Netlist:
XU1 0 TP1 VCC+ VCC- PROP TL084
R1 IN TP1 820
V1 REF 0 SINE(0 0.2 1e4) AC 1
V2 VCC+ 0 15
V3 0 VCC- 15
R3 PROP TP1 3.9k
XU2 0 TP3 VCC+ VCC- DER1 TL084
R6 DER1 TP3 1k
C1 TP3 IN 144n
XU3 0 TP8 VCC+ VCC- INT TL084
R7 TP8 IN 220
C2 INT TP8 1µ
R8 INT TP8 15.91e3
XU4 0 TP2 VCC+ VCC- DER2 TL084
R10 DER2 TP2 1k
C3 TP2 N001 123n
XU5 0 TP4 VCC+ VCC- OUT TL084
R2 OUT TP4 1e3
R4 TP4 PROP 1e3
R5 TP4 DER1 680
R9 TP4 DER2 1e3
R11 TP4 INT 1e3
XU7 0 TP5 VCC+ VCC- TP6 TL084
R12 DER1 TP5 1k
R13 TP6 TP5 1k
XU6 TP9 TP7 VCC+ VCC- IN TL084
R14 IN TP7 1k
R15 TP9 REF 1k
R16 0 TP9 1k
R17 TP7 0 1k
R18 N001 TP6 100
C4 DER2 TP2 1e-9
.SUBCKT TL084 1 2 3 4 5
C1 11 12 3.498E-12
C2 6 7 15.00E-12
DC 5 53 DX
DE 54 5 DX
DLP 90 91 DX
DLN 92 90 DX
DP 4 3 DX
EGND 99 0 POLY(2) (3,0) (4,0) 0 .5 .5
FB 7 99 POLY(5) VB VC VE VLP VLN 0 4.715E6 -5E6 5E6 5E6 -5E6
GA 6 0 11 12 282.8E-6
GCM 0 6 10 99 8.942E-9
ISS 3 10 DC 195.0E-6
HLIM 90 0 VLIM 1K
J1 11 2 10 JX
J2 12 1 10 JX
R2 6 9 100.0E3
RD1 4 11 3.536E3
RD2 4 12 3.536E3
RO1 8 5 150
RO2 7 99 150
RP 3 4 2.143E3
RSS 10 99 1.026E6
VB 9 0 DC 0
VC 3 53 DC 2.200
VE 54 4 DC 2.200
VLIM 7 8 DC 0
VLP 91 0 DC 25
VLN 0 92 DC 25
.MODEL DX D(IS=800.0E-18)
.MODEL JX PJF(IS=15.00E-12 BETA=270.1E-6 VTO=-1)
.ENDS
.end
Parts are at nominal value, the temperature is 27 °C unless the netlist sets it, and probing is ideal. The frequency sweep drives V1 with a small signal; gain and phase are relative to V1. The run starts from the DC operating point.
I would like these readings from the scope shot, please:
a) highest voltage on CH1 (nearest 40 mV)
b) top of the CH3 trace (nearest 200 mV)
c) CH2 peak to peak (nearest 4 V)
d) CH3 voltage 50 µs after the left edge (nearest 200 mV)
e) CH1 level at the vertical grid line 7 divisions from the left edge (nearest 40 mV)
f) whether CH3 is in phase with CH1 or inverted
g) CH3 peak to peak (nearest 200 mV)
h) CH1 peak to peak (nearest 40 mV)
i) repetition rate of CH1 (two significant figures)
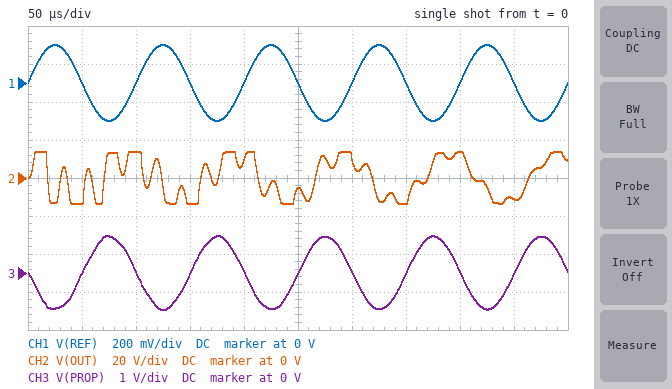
200 mV
1.0 V
28 V
0 V
0 V
inverted
2.0 V
400 mV
10 kHz
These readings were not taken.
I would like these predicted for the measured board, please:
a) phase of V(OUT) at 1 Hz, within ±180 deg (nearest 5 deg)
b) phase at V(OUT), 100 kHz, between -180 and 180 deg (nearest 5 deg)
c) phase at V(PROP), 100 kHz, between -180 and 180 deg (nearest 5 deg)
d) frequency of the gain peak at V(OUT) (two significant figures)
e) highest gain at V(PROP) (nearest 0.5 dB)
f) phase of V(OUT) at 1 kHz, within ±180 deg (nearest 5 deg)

-5 deg
-145 deg
165 deg
46 kHz
26.0 dB
10 deg
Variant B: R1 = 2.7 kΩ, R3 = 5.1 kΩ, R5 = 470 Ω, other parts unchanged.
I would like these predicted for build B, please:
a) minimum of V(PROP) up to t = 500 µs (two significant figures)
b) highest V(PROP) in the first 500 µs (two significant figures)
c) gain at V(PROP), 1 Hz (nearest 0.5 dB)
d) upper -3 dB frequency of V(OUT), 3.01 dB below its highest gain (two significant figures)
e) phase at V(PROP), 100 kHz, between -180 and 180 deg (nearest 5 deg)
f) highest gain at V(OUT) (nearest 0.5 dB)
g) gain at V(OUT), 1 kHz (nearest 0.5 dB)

-390 mV
390 mV
5.5 dB
46 kHz
170 deg
80.0 dB
5.0 dB
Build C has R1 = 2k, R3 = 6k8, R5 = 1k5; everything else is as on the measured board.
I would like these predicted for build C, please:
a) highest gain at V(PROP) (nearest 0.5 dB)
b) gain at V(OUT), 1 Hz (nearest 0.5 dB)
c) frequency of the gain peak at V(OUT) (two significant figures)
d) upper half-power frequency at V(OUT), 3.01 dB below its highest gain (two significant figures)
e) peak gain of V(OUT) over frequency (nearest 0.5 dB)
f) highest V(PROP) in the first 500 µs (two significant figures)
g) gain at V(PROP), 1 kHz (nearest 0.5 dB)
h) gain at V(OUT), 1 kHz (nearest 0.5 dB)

26.5 dB
37.5 dB
47 kHz
48 kHz
83.5 dB
700 mV
10.5 dB
8.5 dB
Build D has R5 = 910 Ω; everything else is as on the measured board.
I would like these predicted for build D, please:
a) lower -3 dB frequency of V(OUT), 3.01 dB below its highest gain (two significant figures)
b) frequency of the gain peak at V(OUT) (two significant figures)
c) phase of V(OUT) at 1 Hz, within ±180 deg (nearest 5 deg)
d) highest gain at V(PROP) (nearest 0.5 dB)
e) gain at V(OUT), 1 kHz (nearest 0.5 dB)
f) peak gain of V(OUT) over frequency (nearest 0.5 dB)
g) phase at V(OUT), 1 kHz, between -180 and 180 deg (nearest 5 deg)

46 kHz
47 kHz
-5 deg
27.5 dB
12.0 dB
82.0 dB
5 deg
